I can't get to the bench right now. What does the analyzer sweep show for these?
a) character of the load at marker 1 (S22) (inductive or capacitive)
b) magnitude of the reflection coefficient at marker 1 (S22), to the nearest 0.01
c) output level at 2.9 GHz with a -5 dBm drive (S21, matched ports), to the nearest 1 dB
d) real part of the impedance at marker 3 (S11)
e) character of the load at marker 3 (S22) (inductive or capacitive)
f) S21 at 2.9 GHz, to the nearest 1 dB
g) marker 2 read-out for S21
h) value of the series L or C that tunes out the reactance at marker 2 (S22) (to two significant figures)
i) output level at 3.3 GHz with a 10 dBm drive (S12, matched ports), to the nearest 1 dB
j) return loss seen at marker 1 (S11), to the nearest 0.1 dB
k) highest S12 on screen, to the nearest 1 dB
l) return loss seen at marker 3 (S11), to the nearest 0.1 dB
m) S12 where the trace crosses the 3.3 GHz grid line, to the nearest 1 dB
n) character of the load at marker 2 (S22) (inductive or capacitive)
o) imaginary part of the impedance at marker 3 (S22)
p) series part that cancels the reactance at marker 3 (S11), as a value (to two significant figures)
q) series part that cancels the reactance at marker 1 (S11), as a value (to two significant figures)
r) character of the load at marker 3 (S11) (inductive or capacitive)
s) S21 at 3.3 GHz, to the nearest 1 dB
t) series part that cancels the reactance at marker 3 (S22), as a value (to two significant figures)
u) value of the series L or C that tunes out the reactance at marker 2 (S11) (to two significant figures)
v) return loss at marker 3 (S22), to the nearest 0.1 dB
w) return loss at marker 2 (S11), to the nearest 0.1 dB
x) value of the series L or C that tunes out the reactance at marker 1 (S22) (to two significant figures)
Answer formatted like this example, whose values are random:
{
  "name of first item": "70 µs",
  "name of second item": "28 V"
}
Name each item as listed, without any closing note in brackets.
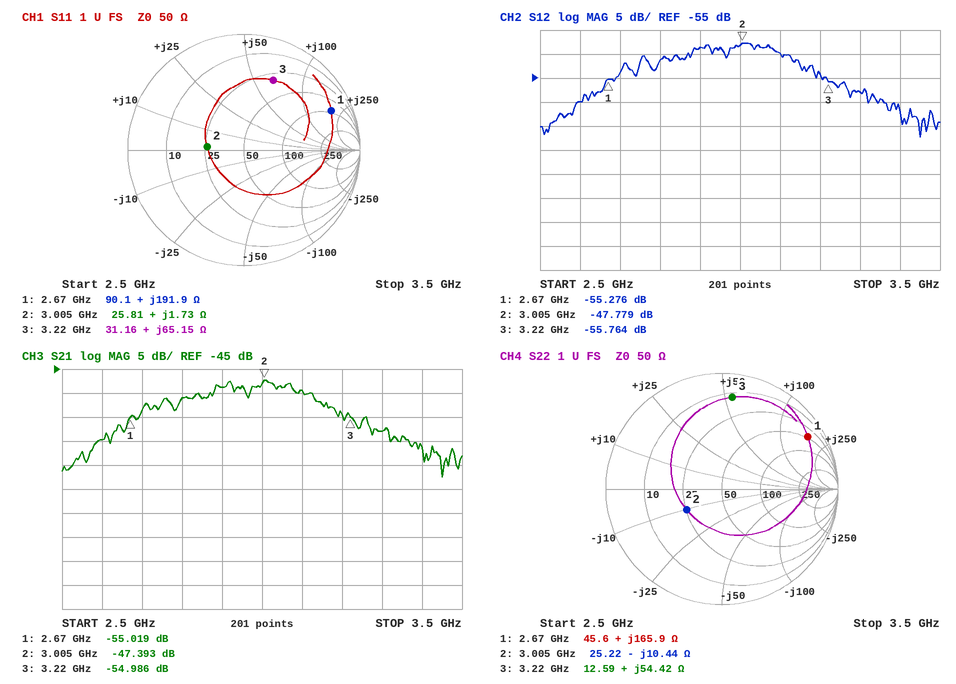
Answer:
{
  "character of the load at marker 1 (S22)": "inductive",
  "magnitude of the reflection coefficient at marker 1 (S22), to the nearest 0.01": "0.87",
  "output level at 2.9 GHz with a -5 dBm drive (S21, matched ports), to the nearest 1 dB": "-54 dBm",
  "real part of the impedance at marker 3": "31.16 Ω",
  "character of the load at marker 3 (S22)": "inductive",
  "S21 at 2.9 GHz, to the nearest 1 dB": "-49 dB",
  "marker 2 read-out for S21": "-47.393 dB",
  "value of the series L or C that tunes out the reactance at marker 2 (S22)": "550 pH",
  "output level at 3.3 GHz with a 10 dBm drive (S12, matched ports), to the nearest 1 dB": "-48 dBm",
  "return loss seen at marker 1 (S11), to the nearest 0.1 dB": "1.7 dB",
  "highest S12 on screen, to the nearest 1 dB": "-48 dB",
  "return loss seen at marker 3 (S11), to the nearest 0.1 dB": "3.7 dB",
  "S12 where the trace crosses the 3.3 GHz grid line, to the nearest 1 dB": "-58 dB",
  "character of the load at marker 2 (S22)": "capacitive",
  "imaginary part of the impedance at marker 3": "+54.42 Ω",
  "series part that cancels the reactance at marker 3 (S11), as a value": "760 fF",
  "series part that cancels the reactance at marker 1 (S11), as a value": "310 fF",
  "character of the load at marker 3 (S11)": "inductive",
  "S21 at 3.3 GHz, to the nearest 1 dB": "-58 dB",
  "series part that cancels the reactance at marker 3 (S22), as a value": "910 fF",
  "value of the series L or C that tunes out the reactance at marker 2 (S11)": "31 pF",
  "return loss at marker 3 (S22), to the nearest 0.1 dB": "2.0 dB",
  "return loss at marker 2 (S11), to the nearest 0.1 dB": "9.9 dB",
  "value of the series L or C that tunes out the reactance at marker 1 (S22)": "360 fF"
}
